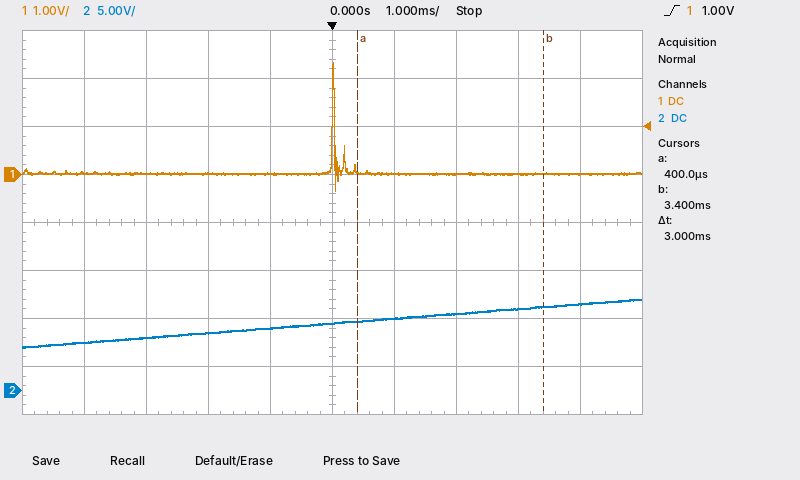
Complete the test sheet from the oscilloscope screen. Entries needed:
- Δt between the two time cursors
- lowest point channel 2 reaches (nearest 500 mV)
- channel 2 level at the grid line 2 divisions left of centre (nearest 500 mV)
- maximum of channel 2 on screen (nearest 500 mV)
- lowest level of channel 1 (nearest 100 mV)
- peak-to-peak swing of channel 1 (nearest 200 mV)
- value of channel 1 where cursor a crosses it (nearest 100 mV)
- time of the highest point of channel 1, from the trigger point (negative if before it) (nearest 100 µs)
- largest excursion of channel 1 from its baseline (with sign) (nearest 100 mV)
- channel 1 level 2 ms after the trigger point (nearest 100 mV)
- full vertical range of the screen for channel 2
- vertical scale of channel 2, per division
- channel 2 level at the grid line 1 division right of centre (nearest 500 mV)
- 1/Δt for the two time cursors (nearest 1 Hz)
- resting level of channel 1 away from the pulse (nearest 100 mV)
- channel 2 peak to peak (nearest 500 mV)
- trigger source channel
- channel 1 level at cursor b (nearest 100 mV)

3 ms
4.5 V
6.0 V
9.5 V
-300 mV
2.6 V
100 mV
0.0 ms
+2.3 V
0.0 V
40 V
5 V
7.5 V
333 Hz
0.0 V
5.0 V
channel 1
0.0 V
